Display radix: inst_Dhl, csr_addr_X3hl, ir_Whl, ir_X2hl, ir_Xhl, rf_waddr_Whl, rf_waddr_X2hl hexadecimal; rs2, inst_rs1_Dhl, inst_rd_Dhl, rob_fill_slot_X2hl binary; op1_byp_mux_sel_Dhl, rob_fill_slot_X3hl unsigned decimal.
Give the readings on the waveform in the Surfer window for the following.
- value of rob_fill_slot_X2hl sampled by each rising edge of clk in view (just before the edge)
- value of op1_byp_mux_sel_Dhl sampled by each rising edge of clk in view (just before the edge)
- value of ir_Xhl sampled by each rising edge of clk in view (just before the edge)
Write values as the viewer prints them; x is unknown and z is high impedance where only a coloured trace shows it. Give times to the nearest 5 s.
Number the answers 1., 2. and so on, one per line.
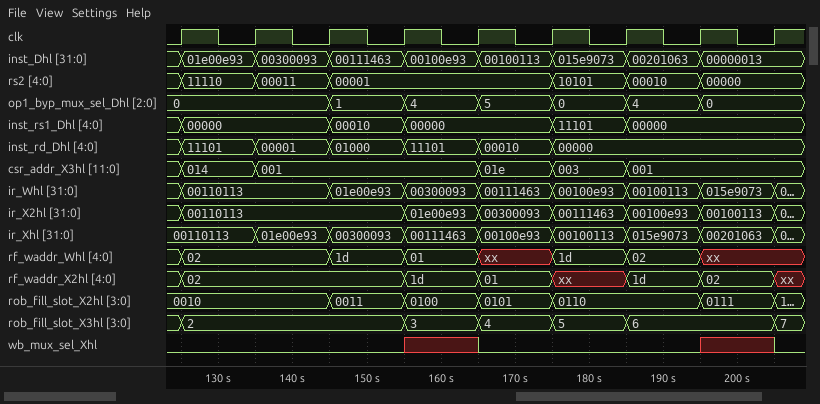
1. 0010, 0010, 0010, 0011, 0100, 0101, 0110, 0110, 0111
2. 0, 0, 0, 1, 4, 5, 0, 4, 0
3. 00110113, 00110113, 01e00e93, 00300093, 00111463, 00100e93, 00100113, 015e9073, 00201063
